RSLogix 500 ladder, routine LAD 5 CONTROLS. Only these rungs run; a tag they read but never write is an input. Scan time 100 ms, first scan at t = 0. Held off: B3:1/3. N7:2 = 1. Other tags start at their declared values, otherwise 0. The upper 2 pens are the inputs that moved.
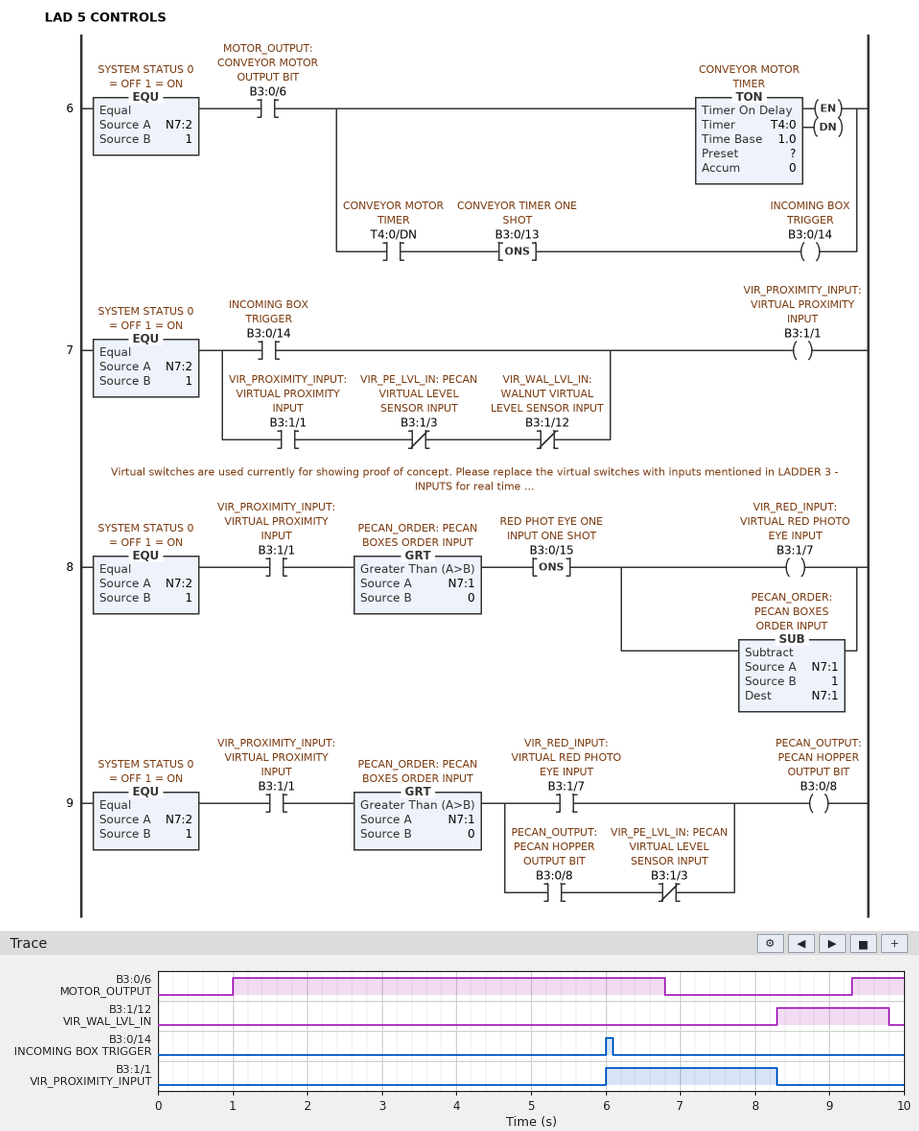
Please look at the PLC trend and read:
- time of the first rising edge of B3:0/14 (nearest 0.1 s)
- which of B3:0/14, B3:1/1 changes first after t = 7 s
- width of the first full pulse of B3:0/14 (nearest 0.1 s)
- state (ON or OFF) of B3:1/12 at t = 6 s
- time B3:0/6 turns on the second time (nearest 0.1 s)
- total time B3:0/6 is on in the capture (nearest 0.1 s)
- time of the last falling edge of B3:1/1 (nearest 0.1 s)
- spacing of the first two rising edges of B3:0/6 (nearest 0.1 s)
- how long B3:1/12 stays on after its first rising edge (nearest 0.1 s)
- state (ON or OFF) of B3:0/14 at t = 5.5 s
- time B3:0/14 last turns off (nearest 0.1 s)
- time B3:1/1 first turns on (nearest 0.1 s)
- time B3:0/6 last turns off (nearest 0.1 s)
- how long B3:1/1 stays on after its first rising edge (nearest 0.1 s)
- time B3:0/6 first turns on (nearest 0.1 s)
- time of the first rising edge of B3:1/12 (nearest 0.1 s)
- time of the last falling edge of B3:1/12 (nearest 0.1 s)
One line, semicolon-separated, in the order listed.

6.0 s; B3:1/1; 0.1 s; OFF; 9.3 s; 6.5 s; 8.3 s; 8.3 s; 1.5 s; OFF; 6.1 s; 6.0 s; 6.8 s; 2.3 s; 1.0 s; 8.3 s; 9.8 s
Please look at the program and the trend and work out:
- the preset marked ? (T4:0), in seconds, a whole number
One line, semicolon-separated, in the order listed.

5 s
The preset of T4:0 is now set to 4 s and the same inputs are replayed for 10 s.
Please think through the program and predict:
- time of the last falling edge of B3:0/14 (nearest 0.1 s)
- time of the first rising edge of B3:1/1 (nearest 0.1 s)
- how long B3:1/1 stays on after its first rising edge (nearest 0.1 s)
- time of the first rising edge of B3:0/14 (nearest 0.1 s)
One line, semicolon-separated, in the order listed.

5.1 s; 5.0 s; 3.3 s; 5.0 s
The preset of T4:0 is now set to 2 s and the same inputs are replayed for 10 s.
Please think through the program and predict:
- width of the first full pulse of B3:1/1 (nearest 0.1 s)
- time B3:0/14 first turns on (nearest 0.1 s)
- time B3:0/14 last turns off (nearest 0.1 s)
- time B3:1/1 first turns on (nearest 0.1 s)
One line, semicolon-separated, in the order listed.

5.3 s; 3.0 s; 3.1 s; 3.0 s
